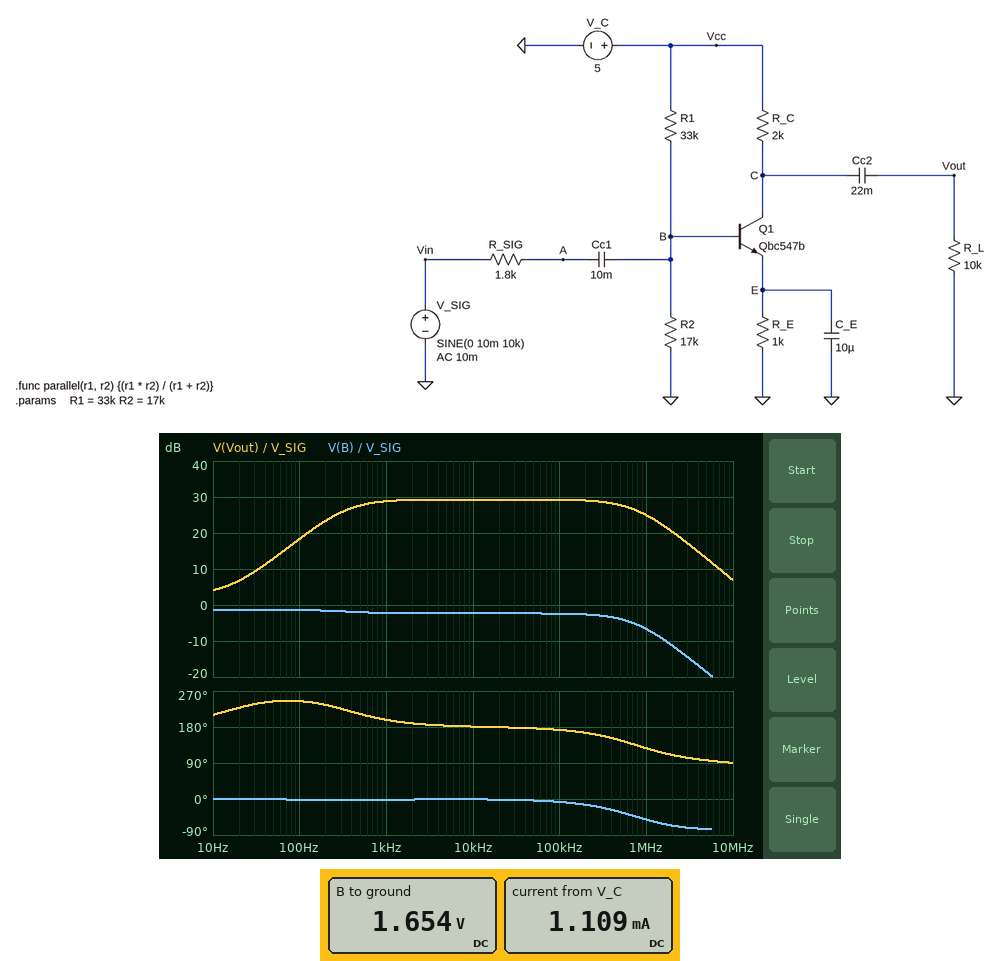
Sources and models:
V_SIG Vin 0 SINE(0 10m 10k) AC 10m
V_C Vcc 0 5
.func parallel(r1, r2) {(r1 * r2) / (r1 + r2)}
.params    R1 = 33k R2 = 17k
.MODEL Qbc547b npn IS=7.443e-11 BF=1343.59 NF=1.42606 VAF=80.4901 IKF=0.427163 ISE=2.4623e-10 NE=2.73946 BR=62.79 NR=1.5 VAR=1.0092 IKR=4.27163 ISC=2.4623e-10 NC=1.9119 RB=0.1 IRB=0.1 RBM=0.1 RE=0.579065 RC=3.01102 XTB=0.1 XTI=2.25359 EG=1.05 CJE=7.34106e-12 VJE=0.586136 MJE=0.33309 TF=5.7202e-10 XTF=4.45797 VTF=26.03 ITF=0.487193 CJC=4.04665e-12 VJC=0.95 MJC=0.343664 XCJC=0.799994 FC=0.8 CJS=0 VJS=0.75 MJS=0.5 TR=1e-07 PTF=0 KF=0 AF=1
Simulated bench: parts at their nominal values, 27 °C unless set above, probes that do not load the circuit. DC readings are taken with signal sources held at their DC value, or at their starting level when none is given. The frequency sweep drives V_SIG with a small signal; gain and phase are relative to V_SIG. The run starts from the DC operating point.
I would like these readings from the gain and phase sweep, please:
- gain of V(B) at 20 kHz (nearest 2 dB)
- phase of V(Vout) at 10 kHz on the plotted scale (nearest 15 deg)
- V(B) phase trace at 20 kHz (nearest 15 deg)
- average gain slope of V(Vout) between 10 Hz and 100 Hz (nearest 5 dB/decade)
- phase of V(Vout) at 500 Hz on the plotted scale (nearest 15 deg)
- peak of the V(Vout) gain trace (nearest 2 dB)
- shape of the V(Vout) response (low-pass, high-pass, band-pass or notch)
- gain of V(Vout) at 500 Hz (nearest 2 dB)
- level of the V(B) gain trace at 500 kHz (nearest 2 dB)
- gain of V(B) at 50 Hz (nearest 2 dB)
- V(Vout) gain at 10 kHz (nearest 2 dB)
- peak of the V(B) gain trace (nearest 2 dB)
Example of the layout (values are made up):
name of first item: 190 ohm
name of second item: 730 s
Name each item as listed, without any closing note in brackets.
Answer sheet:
gain of V(B) at 20 kHz: -2 dB
phase of V(Vout) at 10 kHz on the plotted scale: 180 deg
V(B) phase trace at 20 kHz: 0 deg
average gain slope of V(Vout) between 10 Hz and 100 Hz: 15 dB/decade
phase of V(Vout) at 500 Hz on the plotted scale: 210 deg
peak of the V(Vout) gain trace: 30 dB
shape of the V(Vout) response: band-pass
gain of V(Vout) at 500 Hz: 28 dB
level of the V(B) gain trace at 500 kHz: -4 dB
gain of V(B) at 50 Hz: -2 dB
V(Vout) gain at 10 kHz: 30 dB
peak of the V(B) gain trace: -2 dB
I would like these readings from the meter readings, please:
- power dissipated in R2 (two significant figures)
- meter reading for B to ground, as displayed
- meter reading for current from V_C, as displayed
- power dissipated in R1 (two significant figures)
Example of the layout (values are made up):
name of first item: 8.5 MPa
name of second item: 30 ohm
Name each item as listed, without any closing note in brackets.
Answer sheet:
power dissipated in R2: 160 µW
meter reading for B to ground, as displayed: 1.654 V
meter reading for current from V_C, as displayed: 1.109 mA
power dissipated in R1: 340 µW
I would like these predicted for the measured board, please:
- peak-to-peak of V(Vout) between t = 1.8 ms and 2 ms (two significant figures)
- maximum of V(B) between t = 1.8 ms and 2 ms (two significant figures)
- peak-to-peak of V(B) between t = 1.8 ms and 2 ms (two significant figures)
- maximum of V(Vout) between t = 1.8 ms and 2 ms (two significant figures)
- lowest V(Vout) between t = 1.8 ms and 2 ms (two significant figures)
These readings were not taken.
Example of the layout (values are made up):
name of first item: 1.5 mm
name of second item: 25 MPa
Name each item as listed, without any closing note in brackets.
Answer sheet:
peak-to-peak of V(Vout) between t = 1.8 ms and 2 ms: 580 mV
maximum of V(B) between t = 1.8 ms and 2 ms: 1.7 V
peak-to-peak of V(B) between t = 1.8 ms and 2 ms: 15 mV
maximum of V(Vout) between t = 1.8 ms and 2 ms: 280 mV
lowest V(Vout) between t = 1.8 ms and 2 ms: -300 mV
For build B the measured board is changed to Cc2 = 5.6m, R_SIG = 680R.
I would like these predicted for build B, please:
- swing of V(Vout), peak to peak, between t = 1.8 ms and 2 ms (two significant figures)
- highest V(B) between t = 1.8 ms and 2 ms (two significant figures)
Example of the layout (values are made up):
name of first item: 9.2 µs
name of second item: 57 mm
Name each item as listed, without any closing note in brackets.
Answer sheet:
swing of V(Vout), peak to peak, between t = 1.8 ms and 2 ms: 680 mV
highest V(B) between t = 1.8 ms and 2 ms: 1.7 V
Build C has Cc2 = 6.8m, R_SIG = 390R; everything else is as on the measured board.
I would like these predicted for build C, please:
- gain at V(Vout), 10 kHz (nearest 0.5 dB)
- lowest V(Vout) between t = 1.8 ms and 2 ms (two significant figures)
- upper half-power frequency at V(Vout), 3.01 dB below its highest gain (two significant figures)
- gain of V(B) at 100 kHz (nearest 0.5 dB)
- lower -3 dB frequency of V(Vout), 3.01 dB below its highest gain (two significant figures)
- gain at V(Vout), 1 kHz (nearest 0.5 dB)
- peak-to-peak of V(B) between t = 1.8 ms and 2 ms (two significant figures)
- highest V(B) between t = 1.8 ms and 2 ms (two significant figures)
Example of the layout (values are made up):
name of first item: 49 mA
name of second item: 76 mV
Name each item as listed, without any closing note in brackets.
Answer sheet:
gain at V(Vout), 10 kHz: 31.0 dB
lowest V(Vout) between t = 1.8 ms and 2 ms: -370 mV
upper half-power frequency at V(Vout), 3.01 dB below its highest gain: 2.7 MHz
gain of V(B) at 100 kHz: -0.5 dB
lower -3 dB frequency of V(Vout), 3.01 dB below its highest gain: 370 Hz
gain at V(Vout), 1 kHz: 30.5 dB
peak-to-peak of V(B) between t = 1.8 ms and 2 ms: 19 mV
highest V(B) between t = 1.8 ms and 2 ms: 1.7 V
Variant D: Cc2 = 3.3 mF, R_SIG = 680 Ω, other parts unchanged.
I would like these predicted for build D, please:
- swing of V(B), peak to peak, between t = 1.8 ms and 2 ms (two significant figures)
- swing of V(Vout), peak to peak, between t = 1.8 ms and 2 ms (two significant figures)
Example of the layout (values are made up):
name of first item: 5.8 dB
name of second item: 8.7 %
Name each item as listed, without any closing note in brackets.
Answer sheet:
swing of V(B), peak to peak, between t = 1.8 ms and 2 ms: 18 mV
swing of V(Vout), peak to peak, between t = 1.8 ms and 2 ms: 680 mV
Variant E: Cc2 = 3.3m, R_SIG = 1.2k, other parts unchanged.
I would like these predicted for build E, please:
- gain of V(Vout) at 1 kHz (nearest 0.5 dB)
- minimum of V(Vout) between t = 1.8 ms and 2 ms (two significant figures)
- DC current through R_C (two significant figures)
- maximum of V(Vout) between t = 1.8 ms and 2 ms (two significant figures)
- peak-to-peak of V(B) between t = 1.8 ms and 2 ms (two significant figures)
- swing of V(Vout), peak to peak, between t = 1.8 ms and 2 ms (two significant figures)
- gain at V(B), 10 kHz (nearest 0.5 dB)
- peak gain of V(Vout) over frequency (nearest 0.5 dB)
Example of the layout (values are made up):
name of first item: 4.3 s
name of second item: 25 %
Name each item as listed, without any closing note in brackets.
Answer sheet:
gain of V(Vout) at 1 kHz: 29.5 dB
minimum of V(Vout) between t = 1.8 ms and 2 ms: -330 mV
DC current through R_C: 1.0 mA
maximum of V(Vout) between t = 1.8 ms and 2 ms: 300 mV
peak-to-peak of V(B) between t = 1.8 ms and 2 ms: 17 mV
swing of V(Vout), peak to peak, between t = 1.8 ms and 2 ms: 630 mV
gain at V(B), 10 kHz: -1.5 dB
peak gain of V(Vout) over frequency: 30.0 dB
